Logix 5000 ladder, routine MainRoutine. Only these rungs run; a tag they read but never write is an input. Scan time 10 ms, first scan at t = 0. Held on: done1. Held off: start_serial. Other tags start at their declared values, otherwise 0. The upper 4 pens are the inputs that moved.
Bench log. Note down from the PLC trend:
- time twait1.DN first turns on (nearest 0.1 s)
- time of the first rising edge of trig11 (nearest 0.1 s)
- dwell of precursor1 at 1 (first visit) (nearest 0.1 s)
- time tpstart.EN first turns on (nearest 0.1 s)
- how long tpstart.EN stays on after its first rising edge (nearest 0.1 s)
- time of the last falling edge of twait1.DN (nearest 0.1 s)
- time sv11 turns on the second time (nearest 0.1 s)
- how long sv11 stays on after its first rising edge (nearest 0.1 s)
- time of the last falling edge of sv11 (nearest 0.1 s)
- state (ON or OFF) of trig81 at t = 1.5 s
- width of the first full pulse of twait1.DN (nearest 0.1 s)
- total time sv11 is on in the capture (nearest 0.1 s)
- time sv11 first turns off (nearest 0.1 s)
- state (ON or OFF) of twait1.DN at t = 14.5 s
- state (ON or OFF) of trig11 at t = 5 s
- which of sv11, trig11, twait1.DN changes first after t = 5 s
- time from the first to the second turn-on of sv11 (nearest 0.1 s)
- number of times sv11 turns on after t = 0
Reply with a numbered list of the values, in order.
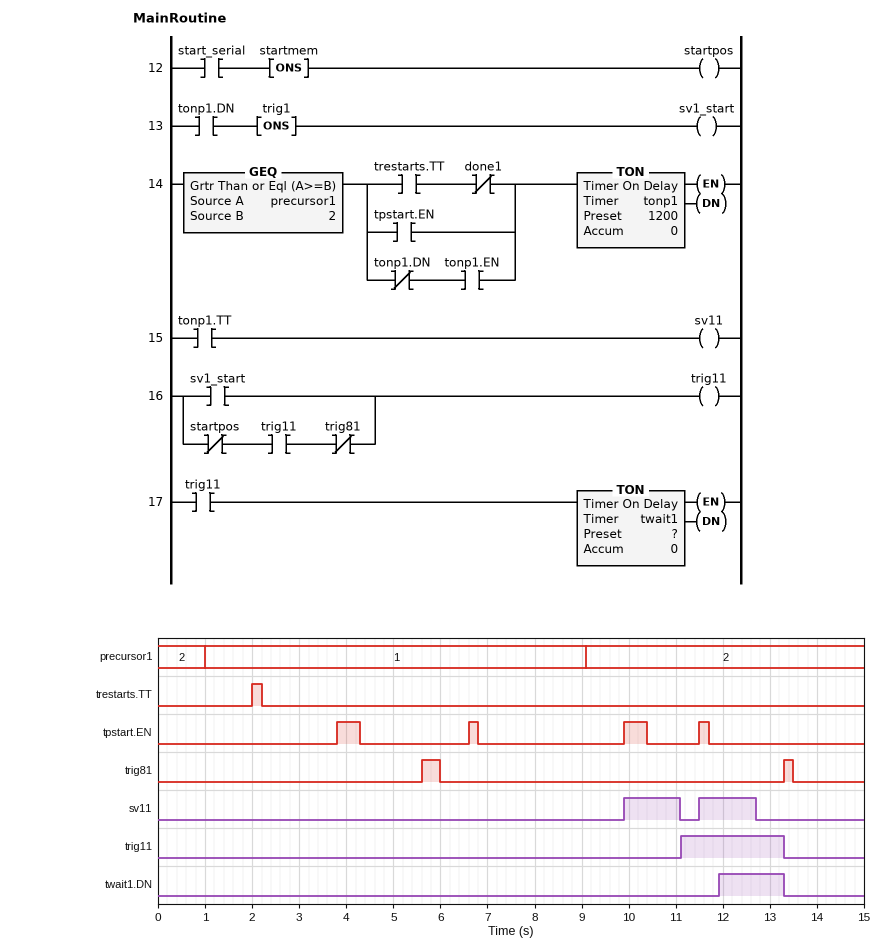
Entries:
1. 11.9 s
2. 11.1 s
3. 8.1 s
4. 3.8 s
5. 0.5 s
6. 13.3 s
7. 11.5 s
8. 1.2 s
9. 12.7 s
10. OFF
11. 1.4 s
12. 2.4 s
13. 11.1 s
14. OFF
15. OFF
16. sv11
17. 1.6 s
18. 2
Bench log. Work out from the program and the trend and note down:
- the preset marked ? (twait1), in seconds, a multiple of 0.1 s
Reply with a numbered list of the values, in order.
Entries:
1. 0.8 s
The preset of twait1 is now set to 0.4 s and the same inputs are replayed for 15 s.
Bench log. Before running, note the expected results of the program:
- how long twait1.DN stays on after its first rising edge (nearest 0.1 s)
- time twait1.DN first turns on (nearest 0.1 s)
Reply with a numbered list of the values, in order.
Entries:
1. 1.8 s
2. 11.5 s
